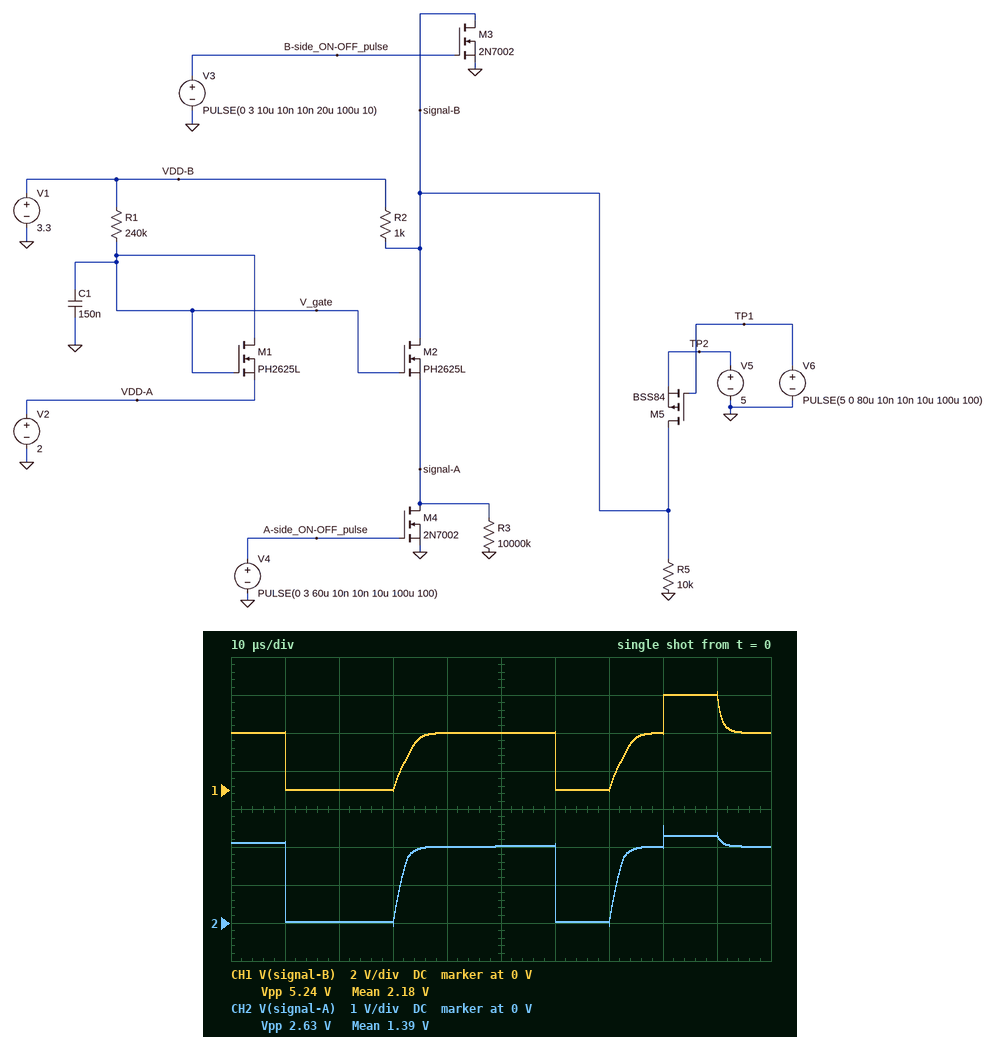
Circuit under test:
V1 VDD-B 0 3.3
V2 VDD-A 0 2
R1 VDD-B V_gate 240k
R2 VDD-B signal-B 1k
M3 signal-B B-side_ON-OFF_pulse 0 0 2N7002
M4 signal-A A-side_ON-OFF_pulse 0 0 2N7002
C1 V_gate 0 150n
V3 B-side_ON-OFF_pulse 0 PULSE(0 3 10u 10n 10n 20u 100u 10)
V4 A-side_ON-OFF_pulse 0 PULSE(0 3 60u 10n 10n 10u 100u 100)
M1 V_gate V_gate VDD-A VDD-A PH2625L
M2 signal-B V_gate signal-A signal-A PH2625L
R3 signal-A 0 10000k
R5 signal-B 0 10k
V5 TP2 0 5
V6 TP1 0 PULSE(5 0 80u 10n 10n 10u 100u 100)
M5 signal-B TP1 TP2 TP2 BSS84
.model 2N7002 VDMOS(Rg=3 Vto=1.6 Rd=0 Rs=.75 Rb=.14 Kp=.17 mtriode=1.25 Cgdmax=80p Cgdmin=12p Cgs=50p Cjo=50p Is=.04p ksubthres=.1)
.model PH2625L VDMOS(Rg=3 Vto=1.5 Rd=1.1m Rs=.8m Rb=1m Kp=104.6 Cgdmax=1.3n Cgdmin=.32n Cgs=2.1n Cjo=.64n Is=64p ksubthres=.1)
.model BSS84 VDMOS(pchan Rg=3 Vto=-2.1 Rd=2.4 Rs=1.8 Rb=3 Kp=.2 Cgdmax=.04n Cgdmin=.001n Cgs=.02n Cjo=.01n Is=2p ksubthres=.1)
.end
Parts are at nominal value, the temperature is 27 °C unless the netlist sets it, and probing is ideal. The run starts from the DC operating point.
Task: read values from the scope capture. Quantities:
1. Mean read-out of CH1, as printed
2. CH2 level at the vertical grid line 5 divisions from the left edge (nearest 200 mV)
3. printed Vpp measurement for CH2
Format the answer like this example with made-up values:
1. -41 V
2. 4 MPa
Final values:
1. 2.18 V
2. 2.0 V
3. 2.63 V
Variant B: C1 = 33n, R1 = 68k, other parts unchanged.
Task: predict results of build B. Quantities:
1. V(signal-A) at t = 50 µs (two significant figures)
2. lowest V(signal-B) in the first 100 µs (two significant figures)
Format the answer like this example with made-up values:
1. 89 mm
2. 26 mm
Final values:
1. 2.1 V
2. -79 mV
